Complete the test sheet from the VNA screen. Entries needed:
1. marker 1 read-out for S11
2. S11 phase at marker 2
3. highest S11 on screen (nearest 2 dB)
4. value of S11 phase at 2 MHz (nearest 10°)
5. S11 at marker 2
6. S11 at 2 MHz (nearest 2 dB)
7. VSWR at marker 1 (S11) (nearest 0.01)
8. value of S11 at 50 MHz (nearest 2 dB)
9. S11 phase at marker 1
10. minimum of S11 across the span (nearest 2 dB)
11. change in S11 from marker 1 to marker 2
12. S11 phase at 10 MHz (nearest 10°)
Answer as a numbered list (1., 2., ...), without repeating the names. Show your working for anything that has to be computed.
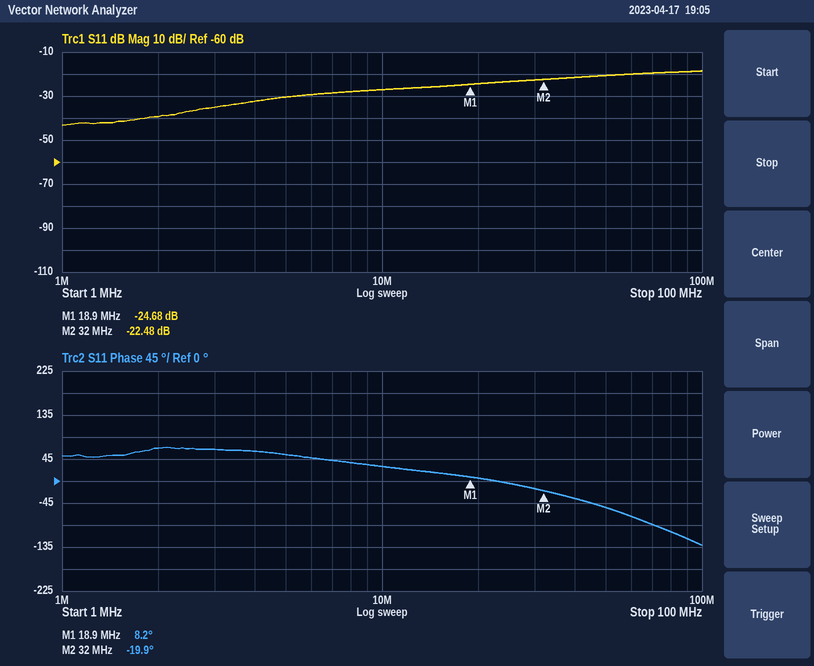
1. -24.68 dB
2. -19.9°
3. -18 dB
4. 70°
5. -22.48 dB
6. -40 dB
7. (1 + 0.0583)/(1 − 0.0583) ≈ 1.12
8. -20 dB
9. 8.2°
10. -44 dB
11. -22.48 − (-24.68) = 2.20 dB
12. 30°
